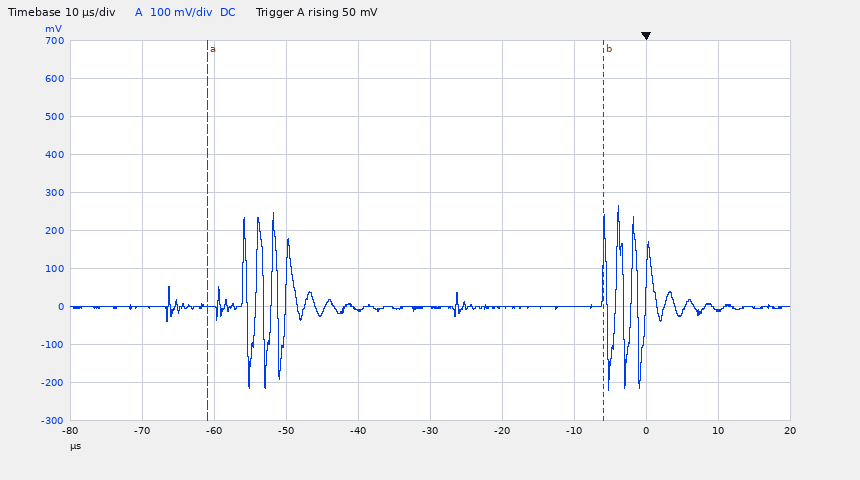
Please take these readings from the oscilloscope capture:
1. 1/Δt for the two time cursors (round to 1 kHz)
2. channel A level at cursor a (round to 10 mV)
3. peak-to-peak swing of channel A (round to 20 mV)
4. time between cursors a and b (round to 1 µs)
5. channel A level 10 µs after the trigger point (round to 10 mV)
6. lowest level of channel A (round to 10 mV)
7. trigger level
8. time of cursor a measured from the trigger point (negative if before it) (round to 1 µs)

18 kHz
0 mV
480 mV
55 µs
-10 mV
-220 mV
50 mV
-61 µs
